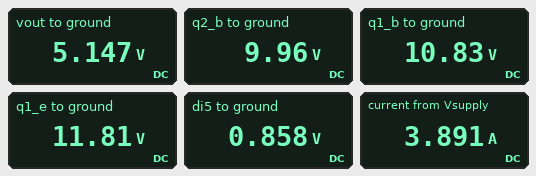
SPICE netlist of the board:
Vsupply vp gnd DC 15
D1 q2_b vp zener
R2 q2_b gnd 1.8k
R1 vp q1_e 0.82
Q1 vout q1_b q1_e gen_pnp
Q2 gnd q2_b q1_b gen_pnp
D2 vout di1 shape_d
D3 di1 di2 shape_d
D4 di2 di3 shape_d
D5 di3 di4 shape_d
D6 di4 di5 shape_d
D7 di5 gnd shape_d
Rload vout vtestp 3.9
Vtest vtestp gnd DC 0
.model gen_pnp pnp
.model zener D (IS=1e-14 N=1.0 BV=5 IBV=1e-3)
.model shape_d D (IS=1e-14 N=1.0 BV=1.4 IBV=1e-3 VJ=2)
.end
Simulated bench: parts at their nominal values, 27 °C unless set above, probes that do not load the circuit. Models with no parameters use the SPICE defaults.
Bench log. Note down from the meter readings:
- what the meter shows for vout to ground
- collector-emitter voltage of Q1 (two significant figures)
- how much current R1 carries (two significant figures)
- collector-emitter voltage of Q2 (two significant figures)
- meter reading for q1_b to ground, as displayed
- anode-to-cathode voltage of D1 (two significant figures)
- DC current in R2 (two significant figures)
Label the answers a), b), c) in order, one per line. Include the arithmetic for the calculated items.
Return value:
a) 5.147 V
b) 5.147 V - 11.81 V = -6.7 V
c) (15 V - 11.81 V) / 820 mΩ = 3.9 A
d) 0 V - 10.83 V = -11 V
e) 10.83 V
f) 9.96 V - 15 V = -5.0 V
g) (9.96 V) / 1.8 kΩ = 5.5 mA
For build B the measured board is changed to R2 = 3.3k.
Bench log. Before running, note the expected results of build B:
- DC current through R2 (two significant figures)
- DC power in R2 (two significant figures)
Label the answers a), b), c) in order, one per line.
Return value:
a) 3.0 mA
b) 30 mW
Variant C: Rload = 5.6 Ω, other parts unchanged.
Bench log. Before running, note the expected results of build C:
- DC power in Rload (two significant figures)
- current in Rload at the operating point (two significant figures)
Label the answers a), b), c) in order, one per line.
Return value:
a) 4.8 W
b) 920 mA
